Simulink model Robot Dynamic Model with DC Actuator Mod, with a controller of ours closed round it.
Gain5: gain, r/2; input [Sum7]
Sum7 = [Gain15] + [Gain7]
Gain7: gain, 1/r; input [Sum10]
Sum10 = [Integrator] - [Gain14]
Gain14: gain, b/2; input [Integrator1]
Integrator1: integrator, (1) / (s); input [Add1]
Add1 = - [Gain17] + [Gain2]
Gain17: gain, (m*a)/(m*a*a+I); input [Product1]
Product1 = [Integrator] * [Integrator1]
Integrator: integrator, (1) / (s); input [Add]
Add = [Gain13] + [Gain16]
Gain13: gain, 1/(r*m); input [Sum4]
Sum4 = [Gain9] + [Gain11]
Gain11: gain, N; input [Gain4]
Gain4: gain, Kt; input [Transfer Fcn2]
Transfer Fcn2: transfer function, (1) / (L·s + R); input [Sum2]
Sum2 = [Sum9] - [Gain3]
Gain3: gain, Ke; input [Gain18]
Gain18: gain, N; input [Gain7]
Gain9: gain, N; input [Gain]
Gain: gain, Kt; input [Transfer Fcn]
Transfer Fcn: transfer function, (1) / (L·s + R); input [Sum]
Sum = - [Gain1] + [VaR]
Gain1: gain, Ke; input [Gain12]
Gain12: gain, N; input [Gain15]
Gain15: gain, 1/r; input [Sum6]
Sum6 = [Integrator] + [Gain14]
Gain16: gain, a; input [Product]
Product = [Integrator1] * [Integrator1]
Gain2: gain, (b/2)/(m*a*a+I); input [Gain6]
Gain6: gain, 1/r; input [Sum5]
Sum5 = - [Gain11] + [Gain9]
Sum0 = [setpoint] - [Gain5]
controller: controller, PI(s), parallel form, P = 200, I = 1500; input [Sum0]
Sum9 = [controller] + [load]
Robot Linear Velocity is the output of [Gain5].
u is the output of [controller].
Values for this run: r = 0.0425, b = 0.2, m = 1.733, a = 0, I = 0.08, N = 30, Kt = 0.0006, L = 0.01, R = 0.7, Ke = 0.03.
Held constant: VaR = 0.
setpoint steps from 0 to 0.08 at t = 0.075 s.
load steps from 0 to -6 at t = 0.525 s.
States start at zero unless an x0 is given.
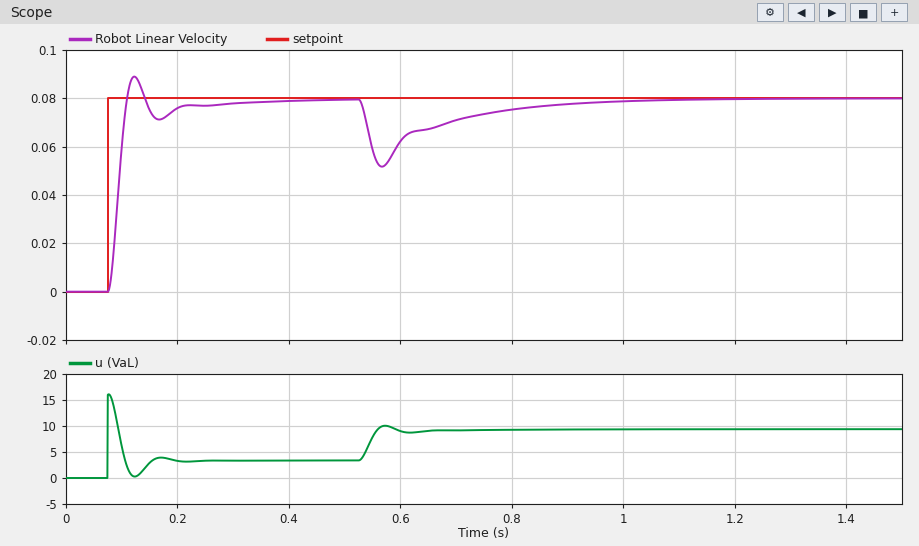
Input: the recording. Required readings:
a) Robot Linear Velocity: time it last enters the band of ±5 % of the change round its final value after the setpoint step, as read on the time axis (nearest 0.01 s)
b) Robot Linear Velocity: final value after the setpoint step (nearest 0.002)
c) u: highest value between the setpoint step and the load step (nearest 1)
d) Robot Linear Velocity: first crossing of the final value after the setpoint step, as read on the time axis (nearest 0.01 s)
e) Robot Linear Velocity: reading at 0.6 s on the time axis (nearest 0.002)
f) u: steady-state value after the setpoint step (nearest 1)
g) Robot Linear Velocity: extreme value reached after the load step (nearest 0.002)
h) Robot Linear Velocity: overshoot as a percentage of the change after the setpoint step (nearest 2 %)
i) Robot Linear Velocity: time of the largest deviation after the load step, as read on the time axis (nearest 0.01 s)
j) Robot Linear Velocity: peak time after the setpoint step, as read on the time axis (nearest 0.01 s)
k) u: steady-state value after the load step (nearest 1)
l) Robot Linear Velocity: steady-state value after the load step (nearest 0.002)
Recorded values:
0.20 s
0.080
16
0.11 s
0.062
3
0.052
12 %
0.57 s
0.12 s
9
0.080
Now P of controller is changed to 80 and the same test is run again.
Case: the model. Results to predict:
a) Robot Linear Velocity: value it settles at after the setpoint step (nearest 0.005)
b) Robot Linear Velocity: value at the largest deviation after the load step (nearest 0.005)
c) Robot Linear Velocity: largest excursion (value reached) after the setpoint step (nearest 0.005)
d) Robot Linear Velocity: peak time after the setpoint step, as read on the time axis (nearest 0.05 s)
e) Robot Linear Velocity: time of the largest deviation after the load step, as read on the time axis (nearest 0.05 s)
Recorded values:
0.080
0.035
0.085
0.15 s
0.60 s
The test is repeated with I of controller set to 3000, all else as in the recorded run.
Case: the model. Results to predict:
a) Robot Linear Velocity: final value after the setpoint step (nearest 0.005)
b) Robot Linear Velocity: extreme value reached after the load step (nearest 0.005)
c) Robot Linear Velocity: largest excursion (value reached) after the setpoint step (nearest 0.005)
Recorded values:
0.080
0.055
0.100
